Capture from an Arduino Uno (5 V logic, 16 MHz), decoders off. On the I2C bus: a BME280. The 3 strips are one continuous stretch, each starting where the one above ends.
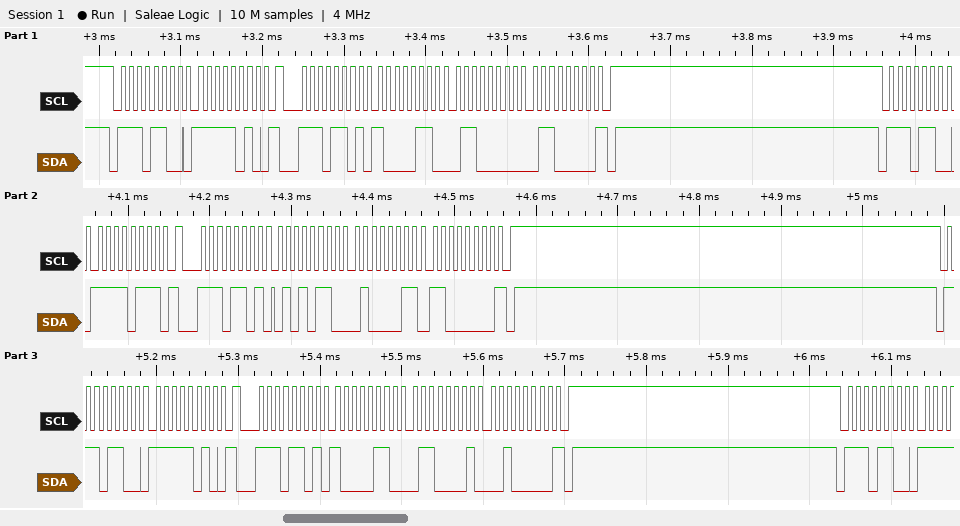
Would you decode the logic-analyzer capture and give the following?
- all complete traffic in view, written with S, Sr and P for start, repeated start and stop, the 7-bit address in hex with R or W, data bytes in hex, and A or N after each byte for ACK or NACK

S 76W A FA A Sr 76R A 86 A 60 A 60 N P S 76W A F7 A Sr 76R A 56 A 43 A C0 N P S 76W A FA A Sr 76R A 86 A 61 A 20 N P S 76W A
